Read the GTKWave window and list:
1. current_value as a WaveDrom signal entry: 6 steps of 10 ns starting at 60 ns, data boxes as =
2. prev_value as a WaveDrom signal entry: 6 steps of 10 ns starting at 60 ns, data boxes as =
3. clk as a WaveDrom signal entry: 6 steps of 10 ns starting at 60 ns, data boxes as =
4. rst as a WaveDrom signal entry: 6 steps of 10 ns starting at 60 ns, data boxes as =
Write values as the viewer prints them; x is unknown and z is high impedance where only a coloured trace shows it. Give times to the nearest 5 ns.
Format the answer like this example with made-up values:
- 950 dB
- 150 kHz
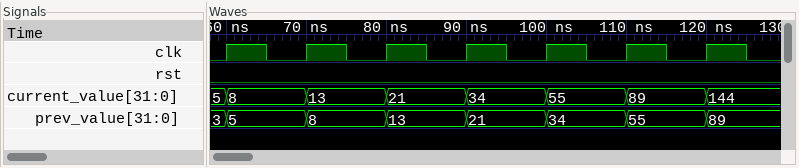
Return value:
- {name: 'current_value', wave: '======', data: '8 13 21 34 55 89'}
- {name: 'prev_value', wave: '======', data: '5 8 13 21 34 55'}
- {name: 'clk', wave: 'p.....'}
- {name: 'rst', wave: '0.....'}
